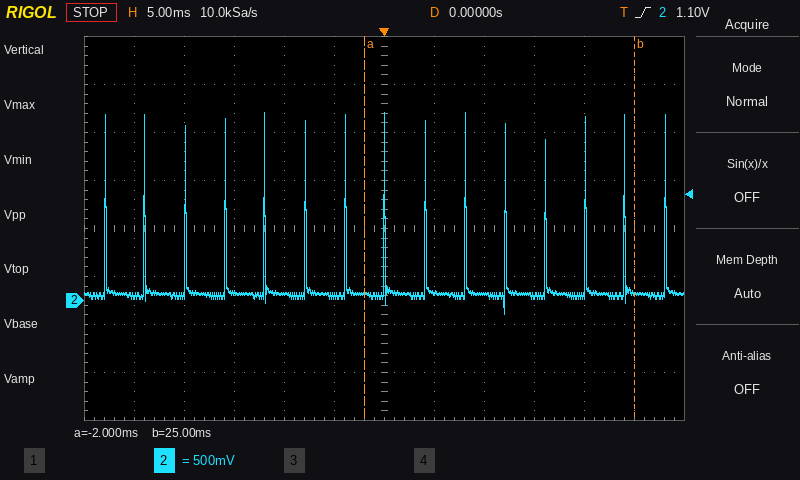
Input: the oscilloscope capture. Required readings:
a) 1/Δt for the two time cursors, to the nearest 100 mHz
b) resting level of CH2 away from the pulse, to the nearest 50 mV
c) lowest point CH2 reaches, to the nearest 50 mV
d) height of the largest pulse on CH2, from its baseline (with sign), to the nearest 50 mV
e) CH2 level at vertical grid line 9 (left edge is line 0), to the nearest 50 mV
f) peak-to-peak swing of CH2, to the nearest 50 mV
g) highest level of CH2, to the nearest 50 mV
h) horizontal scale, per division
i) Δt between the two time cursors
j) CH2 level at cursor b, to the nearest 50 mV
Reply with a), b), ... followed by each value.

a) 37.0 Hz
b) 50 mV
c) -150 mV
d) +1.90 V
e) 50 mV
f) 2.10 V
g) 1.95 V
h) 5 ms
i) 27.0 ms
j) 100 mV
